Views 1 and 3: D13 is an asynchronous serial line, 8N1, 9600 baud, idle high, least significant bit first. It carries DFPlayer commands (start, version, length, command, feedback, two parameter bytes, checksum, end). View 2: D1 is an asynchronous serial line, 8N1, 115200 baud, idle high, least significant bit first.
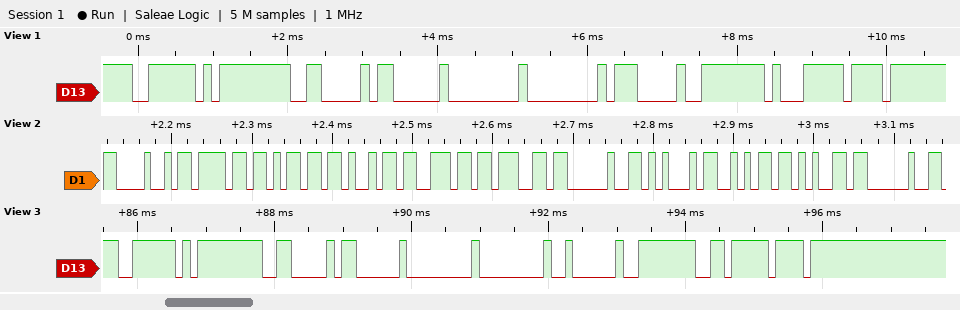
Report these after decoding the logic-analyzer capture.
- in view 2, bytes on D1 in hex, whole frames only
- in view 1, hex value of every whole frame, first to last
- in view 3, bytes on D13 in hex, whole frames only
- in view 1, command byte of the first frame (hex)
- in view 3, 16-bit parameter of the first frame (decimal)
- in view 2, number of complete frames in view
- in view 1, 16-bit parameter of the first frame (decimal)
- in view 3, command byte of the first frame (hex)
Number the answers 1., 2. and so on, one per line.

1. 0x48 0x6F 0x6D 0x69 0x6E 0x67 0x20 0x45 0x6A 0x65 0x20
2. 7E FF 06 03 00 00 07 FE F1 EF
3. 7E FF 06 03 00 00 02 FE F6 EF
4. 0x03
5. 2
6. 11
7. 7
8. 0x03
